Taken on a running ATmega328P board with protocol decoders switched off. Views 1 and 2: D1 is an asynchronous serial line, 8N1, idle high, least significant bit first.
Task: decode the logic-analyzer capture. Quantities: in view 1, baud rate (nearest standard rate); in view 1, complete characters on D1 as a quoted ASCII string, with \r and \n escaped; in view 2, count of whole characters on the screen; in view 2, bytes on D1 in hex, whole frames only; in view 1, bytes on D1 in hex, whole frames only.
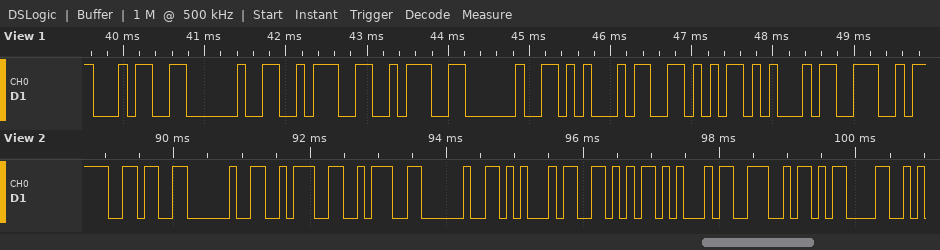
9600 baud
"4 :: EVEN"
10
36 20 3A 3A 20 45 56 45 4E 0D
0x34 0x20 0x3A 0x3A 0x20 0x45 0x56 0x45 0x4E
